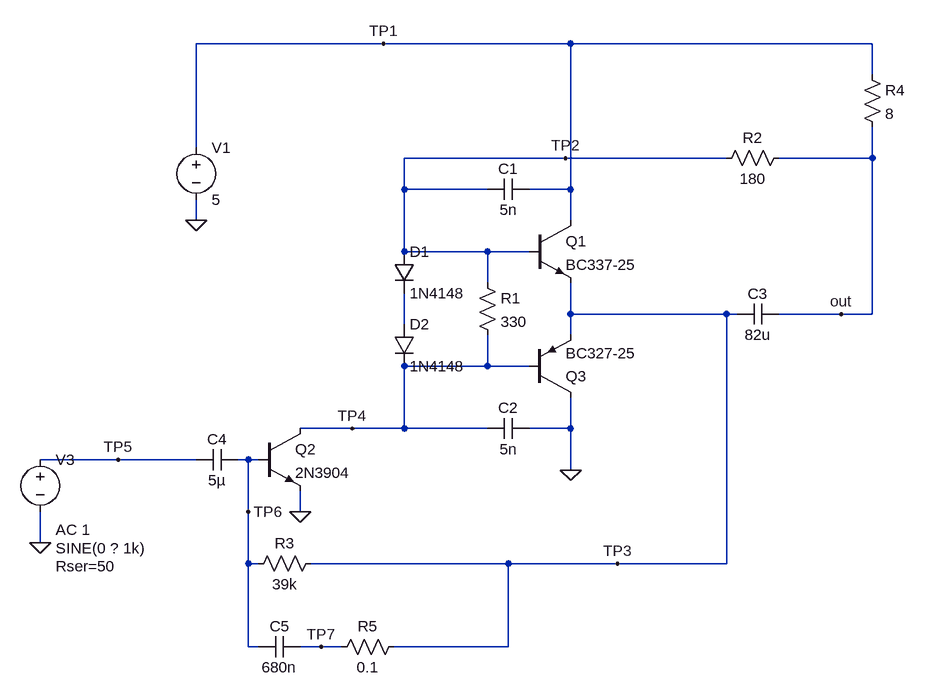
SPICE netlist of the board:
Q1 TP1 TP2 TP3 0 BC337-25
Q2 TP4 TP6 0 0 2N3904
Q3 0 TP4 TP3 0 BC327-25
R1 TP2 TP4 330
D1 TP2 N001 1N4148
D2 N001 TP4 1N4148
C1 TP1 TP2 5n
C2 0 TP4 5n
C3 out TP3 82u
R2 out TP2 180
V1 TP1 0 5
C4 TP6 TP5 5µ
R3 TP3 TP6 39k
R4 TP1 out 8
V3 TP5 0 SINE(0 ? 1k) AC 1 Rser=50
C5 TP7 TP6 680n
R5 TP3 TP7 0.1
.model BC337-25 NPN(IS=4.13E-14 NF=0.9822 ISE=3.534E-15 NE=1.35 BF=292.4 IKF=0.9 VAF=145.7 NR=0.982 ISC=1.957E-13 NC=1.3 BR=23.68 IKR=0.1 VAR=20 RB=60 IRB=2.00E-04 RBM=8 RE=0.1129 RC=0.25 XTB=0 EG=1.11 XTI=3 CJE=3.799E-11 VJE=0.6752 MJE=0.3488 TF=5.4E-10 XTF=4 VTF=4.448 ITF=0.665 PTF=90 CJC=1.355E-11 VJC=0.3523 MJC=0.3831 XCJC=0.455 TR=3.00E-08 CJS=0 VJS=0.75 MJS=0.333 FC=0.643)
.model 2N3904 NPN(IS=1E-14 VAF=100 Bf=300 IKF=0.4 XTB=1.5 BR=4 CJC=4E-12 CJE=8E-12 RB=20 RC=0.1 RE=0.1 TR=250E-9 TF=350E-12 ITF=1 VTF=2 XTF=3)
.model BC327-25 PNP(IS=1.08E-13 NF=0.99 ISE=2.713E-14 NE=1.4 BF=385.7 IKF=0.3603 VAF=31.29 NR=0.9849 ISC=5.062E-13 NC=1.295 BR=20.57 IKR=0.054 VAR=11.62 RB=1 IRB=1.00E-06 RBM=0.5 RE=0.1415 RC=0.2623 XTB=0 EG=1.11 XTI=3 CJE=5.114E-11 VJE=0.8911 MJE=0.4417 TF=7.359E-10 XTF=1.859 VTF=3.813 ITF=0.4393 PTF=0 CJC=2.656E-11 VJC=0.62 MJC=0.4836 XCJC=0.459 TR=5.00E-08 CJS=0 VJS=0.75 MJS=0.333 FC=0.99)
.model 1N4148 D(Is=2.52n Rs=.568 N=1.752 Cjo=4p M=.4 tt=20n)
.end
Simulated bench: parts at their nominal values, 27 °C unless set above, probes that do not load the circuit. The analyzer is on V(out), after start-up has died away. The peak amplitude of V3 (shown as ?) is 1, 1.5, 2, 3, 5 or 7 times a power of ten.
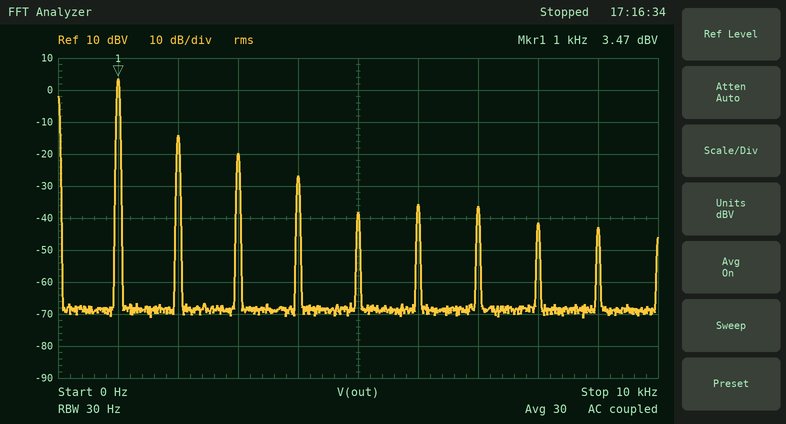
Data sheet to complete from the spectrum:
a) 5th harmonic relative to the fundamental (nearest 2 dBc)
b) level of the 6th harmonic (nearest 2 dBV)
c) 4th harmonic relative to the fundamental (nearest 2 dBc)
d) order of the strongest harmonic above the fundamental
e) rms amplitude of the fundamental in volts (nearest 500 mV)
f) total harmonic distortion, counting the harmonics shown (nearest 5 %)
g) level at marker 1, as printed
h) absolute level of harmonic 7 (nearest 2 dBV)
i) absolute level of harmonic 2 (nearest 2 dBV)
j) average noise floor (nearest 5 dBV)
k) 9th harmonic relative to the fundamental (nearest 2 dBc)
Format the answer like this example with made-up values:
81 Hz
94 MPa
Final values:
-42 dBc
-36 dBV
-30 dBc
2
1.5 V
15 %
3.47 dBV
-36 dBV
-14 dBV
-70 dBV
-46 dBc
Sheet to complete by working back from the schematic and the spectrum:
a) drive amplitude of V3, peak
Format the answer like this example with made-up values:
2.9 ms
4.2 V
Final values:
700 mV
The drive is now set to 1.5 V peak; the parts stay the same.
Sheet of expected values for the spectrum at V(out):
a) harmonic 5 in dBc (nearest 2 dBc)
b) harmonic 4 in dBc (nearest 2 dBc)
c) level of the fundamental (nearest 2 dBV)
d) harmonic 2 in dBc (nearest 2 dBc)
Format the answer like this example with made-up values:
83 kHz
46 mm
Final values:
-30 dBc
-22 dBc
2 dBV
-6 dBc
